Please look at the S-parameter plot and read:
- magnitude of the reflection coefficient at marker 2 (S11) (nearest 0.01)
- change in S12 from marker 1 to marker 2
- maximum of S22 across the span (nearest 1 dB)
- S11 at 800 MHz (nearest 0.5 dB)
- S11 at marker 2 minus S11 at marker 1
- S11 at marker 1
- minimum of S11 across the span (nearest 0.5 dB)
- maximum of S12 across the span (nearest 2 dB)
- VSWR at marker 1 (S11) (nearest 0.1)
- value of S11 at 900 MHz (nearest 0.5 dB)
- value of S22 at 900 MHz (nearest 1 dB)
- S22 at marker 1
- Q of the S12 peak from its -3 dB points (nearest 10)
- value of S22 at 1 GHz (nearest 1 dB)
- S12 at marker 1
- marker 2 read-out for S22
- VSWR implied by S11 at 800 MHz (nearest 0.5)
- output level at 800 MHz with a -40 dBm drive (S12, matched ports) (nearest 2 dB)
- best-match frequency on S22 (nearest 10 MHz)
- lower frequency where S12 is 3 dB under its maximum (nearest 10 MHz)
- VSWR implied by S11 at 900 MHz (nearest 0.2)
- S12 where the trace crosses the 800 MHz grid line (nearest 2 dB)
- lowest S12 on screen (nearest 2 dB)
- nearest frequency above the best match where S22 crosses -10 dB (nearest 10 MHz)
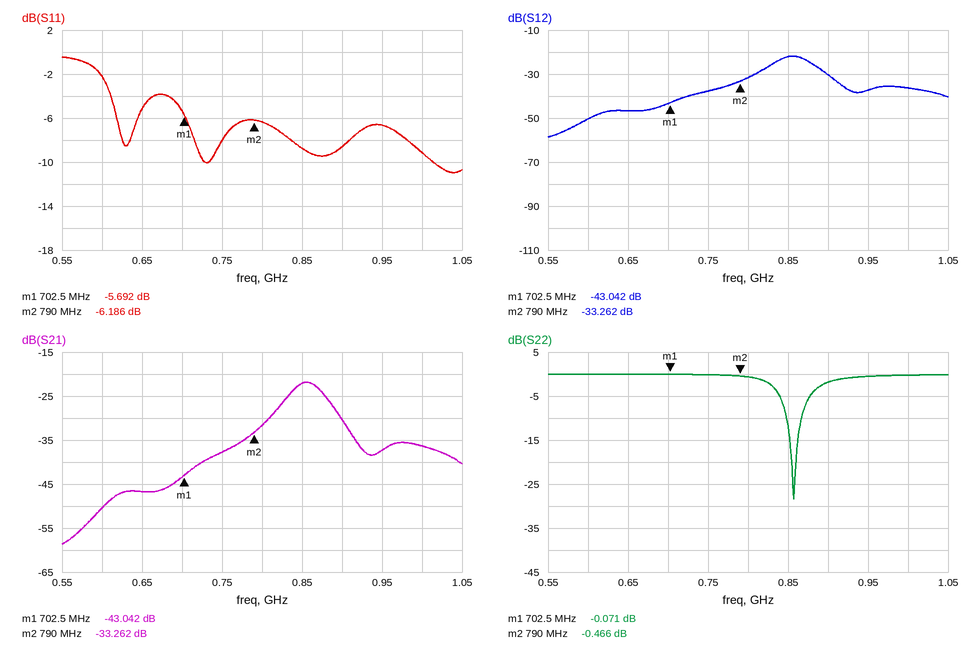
0.49
9.780 dB
0 dB
-6.5 dB
-0.494 dB
-5.692 dB
-11.0 dB
-22 dB
3.2
-8.5 dB
-2 dB
-0.071 dB
20
0 dB
-43.042 dB
-0.466 dB
3.0
-72 dBm
860 MHz
830 MHz
2.2
-32 dB
-58 dB
870 MHz
